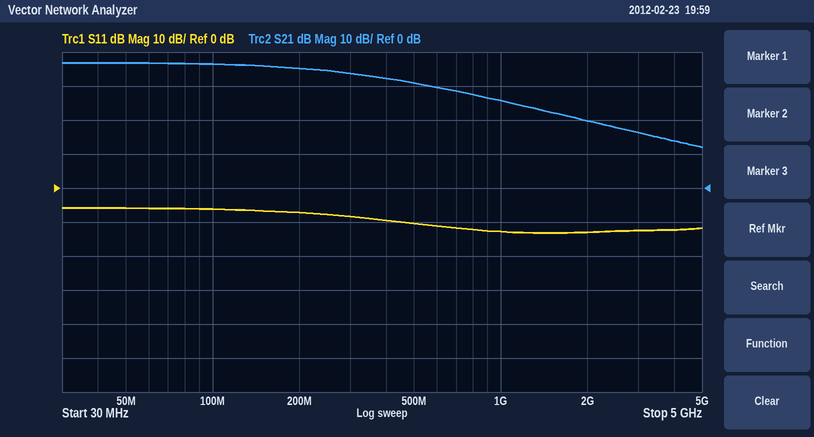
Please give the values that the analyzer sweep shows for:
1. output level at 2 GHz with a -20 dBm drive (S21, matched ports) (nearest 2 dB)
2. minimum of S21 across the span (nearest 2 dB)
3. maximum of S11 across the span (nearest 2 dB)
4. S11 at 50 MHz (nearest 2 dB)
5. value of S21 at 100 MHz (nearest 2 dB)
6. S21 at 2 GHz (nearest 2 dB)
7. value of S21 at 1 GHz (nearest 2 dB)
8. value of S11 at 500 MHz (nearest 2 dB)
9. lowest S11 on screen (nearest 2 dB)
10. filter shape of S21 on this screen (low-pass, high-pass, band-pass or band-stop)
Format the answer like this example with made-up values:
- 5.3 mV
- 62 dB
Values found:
- 0 dBm
- 12 dB
- -6 dB
- -6 dB
- 36 dB
- 20 dB
- 26 dB
- -10 dB
- -14 dB
- low-pass
